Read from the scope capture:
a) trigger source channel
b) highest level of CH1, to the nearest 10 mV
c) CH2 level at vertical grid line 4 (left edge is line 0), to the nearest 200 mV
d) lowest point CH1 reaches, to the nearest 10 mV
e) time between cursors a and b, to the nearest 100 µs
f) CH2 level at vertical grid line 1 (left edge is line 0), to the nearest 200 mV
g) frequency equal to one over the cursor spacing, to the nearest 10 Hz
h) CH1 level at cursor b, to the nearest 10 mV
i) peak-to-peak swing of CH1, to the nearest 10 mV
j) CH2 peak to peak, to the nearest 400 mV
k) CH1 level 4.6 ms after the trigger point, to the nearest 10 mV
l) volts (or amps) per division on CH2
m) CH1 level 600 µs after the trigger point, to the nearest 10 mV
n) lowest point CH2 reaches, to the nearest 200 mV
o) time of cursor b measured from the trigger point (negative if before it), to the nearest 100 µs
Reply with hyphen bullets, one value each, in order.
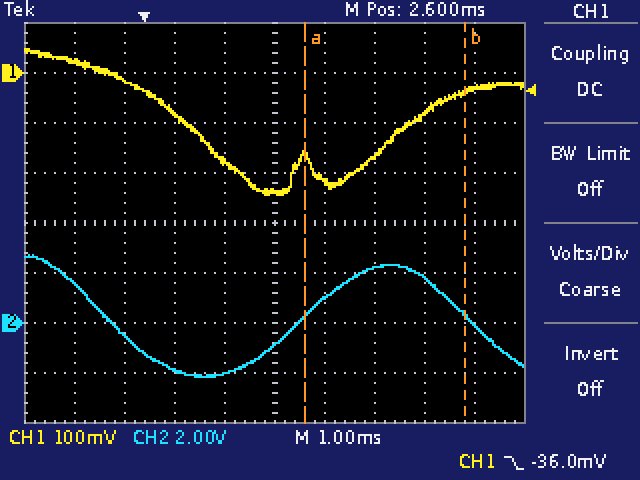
- CH1
- 50 mV
- -2.0 V
- -240 mV
- 3.2 ms
- 1.6 V
- 310 Hz
- -40 mV
- 290 mV
- 4.8 V
- -170 mV
- 2 V
- -80 mV
- -2.2 V
- +6.4 ms
